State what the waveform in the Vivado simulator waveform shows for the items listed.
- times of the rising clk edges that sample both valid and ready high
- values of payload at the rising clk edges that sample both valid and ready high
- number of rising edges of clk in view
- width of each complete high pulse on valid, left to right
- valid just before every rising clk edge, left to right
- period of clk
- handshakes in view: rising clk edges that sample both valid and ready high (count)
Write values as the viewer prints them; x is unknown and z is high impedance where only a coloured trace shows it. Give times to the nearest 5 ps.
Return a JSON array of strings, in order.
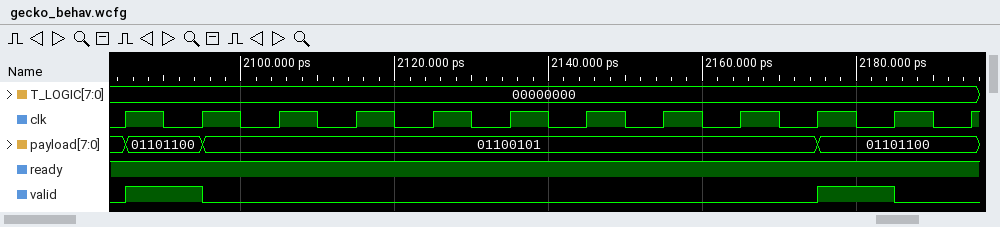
["2095 ps, 2185 ps", "01101100, 01101100", "12", "10 ps, 10 ps", "0 1 0 0 0 0 0 0 0 0 1 0", "10 ps", "2"]
